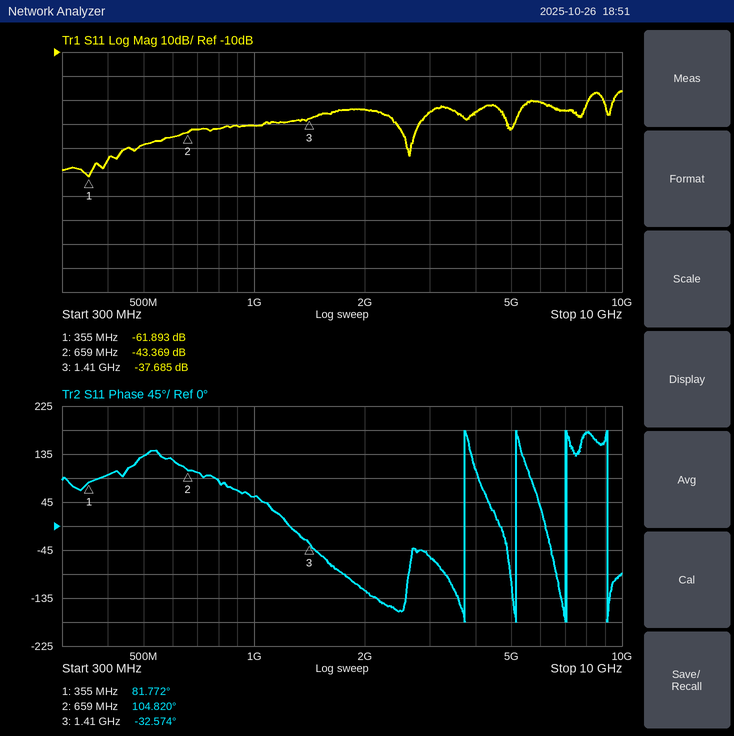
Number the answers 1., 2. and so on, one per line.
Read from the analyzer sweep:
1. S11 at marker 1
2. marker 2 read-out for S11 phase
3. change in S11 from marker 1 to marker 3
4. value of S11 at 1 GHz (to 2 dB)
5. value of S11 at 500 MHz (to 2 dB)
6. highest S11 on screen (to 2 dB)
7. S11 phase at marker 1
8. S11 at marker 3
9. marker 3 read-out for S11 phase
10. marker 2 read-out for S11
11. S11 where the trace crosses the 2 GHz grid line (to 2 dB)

1. -61.893 dB
2. 104.820°
3. 24.208 dB
4. -40 dB
5. -48 dB
6. -26 dB
7. 81.772°
8. -37.685 dB
9. -32.574°
10. -43.369 dB
11. -34 dB
